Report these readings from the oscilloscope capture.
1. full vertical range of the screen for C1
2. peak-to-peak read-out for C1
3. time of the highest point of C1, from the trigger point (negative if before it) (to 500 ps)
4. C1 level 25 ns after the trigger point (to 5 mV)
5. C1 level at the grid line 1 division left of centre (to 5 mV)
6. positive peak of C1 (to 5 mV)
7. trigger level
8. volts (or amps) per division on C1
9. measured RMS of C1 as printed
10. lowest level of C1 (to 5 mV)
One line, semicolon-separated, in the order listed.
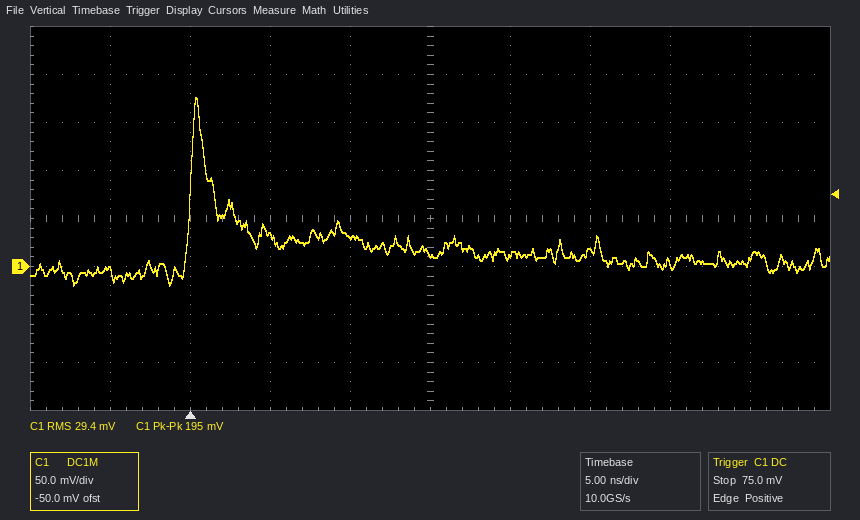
400 mV; 195 mV; +500 ps; 15 mV; 30 mV; 175 mV; 75.0 mV; 50 mV; 29.4 mV; -20 mV
